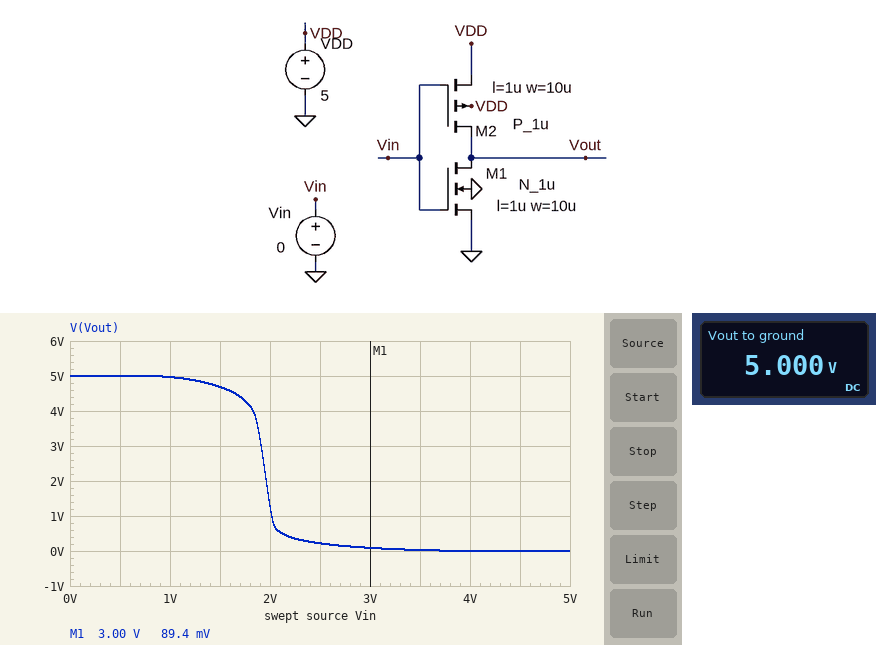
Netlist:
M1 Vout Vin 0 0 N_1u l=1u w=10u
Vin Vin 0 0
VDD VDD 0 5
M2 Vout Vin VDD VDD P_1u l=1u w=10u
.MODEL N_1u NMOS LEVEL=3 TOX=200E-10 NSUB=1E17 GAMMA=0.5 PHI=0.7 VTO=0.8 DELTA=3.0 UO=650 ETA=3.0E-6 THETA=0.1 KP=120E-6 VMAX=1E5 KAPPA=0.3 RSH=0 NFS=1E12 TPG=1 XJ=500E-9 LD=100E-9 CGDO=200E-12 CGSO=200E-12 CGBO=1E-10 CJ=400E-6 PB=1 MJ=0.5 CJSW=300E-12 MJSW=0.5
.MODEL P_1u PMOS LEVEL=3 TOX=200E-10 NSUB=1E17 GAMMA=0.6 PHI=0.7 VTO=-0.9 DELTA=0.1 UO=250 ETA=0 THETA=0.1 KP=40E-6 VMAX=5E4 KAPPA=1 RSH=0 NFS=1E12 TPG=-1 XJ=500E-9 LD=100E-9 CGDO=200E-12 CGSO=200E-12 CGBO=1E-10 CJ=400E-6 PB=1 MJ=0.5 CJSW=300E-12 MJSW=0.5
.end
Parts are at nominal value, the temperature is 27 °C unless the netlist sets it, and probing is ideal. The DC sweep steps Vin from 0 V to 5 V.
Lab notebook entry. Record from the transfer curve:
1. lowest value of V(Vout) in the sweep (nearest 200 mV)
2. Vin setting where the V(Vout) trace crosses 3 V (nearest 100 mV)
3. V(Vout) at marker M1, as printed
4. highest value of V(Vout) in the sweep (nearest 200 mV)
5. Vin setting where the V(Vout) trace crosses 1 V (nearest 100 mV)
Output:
0 V
1.9 V
89.4 mV
5.0 V
2.0 V
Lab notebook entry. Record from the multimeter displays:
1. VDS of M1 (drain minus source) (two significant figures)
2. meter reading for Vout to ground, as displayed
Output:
5.0 V
5.000 V
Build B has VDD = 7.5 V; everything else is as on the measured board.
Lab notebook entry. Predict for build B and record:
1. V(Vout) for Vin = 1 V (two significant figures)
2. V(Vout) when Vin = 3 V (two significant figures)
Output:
7.5 V
1.1 V
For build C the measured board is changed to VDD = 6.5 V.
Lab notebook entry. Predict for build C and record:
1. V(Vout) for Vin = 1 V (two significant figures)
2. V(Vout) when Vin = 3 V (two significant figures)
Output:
6.5 V
420 mV
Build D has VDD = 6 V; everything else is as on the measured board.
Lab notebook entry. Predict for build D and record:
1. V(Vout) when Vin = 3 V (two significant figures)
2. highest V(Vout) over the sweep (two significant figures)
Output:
280 mV
6.0 V
